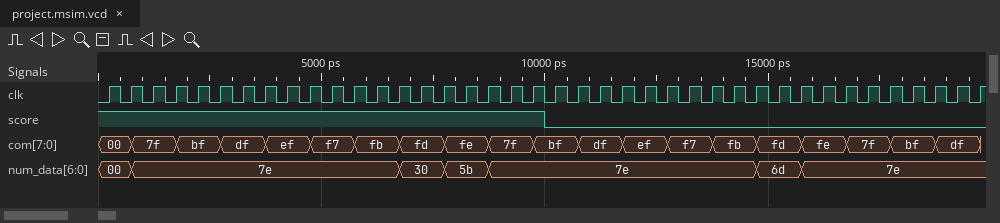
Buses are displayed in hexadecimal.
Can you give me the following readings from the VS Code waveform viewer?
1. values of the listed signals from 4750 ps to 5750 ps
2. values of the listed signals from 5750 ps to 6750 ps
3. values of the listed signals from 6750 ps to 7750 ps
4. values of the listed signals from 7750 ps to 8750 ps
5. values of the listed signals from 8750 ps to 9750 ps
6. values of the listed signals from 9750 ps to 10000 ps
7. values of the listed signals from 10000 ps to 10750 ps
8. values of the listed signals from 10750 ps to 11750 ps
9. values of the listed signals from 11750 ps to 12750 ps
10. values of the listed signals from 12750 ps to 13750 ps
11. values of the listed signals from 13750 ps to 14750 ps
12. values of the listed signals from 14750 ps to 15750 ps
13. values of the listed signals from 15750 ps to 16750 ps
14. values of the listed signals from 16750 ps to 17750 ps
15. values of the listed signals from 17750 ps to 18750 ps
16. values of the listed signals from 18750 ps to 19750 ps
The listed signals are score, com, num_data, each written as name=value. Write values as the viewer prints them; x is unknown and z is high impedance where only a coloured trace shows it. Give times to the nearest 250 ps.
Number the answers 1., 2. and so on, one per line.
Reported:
1. score=1, com=f7, num_data=7e
2. score=1, com=fb, num_data=7e
3. score=1, com=fd, num_data=30
4. score=1, com=fe, num_data=5b
5. score=1, com=7f, num_data=7e
6. score=1, com=bf, num_data=7e
7. score=0, com=bf, num_data=7e
8. score=0, com=df, num_data=7e
9. score=0, com=ef, num_data=7e
10. score=0, com=f7, num_data=7e
11. score=0, com=fb, num_data=7e
12. score=0, com=fd, num_data=6d
13. score=0, com=fe, num_data=7e
14. score=0, com=7f, num_data=7e
15. score=0, com=bf, num_data=7e
16. score=0, com=df, num_data=7e
